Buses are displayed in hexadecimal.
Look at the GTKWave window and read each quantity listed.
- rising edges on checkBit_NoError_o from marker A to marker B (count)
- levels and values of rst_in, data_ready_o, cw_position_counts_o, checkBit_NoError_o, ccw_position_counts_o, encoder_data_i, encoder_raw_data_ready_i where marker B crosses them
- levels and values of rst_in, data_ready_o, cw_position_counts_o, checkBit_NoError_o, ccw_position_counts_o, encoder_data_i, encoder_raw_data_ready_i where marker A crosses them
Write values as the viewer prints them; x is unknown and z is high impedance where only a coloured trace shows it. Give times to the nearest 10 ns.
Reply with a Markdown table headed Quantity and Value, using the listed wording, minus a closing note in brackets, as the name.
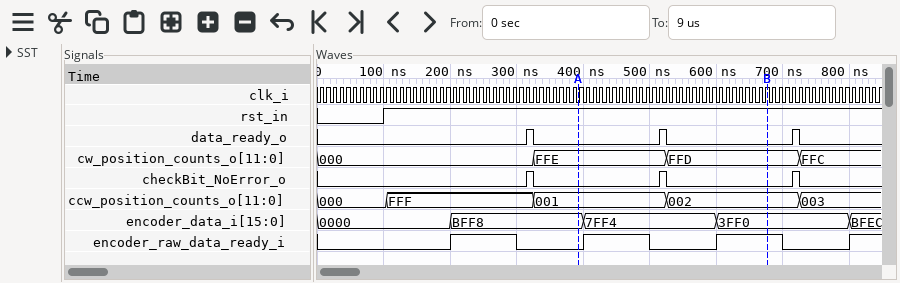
| Quantity | Value |
|---|---|
| rising edges on checkBit_NoError_o from marker A to marker B | 1 |
| levels and values of rst_in, data_ready_o, cw_position_counts_o, checkBit_NoError_o, ccw_position_counts_o, encoder_data_i, encoder_raw_data_ready_i where marker B crosses them | rst_in=1, data_ready_o=0, cw_position_counts_o=FFD, checkBit_NoError_o=0, ccw_position_counts_o=002, encoder_data_i=3FF0, encoder_raw_data_ready_i=1 |
| levels and values of rst_in, data_ready_o, cw_position_counts_o, checkBit_NoError_o, ccw_position_counts_o, encoder_data_i, encoder_raw_data_ready_i where marker A crosses them | rst_in=1, data_ready_o=0, cw_position_counts_o=FFE, checkBit_NoError_o=0, ccw_position_counts_o=001, encoder_data_i=BFF8, encoder_raw_data_ready_i=0 |
